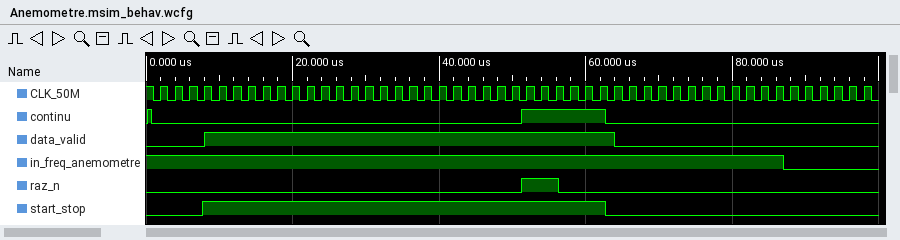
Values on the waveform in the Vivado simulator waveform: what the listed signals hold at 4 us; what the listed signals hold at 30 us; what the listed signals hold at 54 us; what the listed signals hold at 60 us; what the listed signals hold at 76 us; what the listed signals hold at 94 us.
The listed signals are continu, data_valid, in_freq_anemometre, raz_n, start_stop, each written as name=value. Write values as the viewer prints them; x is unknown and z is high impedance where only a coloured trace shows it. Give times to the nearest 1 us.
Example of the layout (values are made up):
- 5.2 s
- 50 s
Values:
- continu=0, data_valid=0, in_freq_anemometre=1, raz_n=0, start_stop=0
- continu=0, data_valid=1, in_freq_anemometre=1, raz_n=0, start_stop=1
- continu=1, data_valid=1, in_freq_anemometre=1, raz_n=1, start_stop=1
- continu=1, data_valid=1, in_freq_anemometre=1, raz_n=0, start_stop=1
- continu=0, data_valid=0, in_freq_anemometre=1, raz_n=0, start_stop=0
- continu=0, data_valid=0, in_freq_anemometre=0, raz_n=0, start_stop=0
